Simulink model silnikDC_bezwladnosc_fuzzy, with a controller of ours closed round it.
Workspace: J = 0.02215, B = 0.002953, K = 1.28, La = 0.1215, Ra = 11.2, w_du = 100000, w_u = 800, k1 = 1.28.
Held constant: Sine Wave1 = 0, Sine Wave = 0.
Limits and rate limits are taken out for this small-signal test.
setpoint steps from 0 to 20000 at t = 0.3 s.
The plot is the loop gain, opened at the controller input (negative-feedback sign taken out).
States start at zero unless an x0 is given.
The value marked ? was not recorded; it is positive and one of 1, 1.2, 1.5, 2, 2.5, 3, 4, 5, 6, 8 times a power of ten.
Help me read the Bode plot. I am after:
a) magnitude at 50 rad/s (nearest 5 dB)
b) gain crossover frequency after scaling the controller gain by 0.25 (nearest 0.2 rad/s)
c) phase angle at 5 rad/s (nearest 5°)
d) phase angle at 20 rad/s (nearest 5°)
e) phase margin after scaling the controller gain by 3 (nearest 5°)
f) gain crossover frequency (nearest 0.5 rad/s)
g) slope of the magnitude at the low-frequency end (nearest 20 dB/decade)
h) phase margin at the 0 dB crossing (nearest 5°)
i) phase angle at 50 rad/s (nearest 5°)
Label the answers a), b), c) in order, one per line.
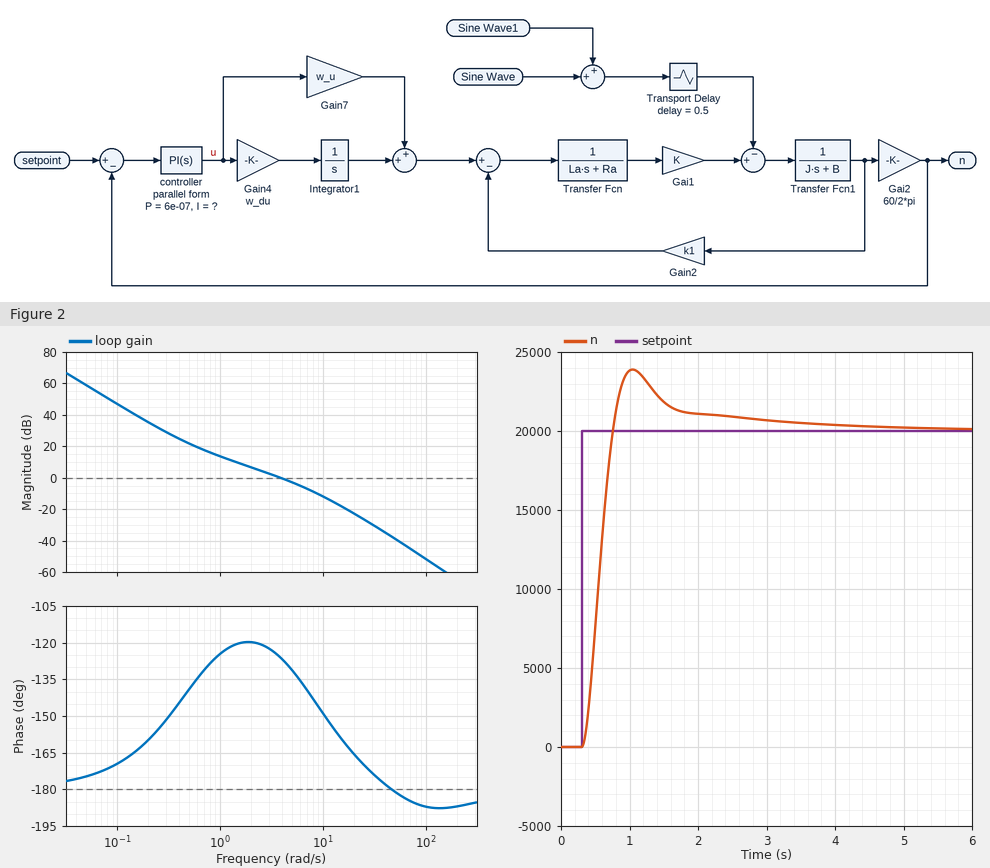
a) -40 dB
b) 1.2 rad/s
c) -130°
d) -165°
e) 35°
f) 4.0 rad/s
g) -40 dB/decade
h) 55°
i) -180°
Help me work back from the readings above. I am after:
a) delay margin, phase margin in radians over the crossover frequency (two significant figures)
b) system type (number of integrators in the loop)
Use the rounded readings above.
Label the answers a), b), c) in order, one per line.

a) 0.24 s
b) 2
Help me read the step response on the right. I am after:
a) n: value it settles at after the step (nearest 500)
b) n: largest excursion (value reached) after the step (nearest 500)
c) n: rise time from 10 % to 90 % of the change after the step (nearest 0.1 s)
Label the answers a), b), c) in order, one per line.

a) 20000
b) 24000
c) 0.3 s
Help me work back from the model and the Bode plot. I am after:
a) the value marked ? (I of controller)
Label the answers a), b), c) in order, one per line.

a) 3e-07
